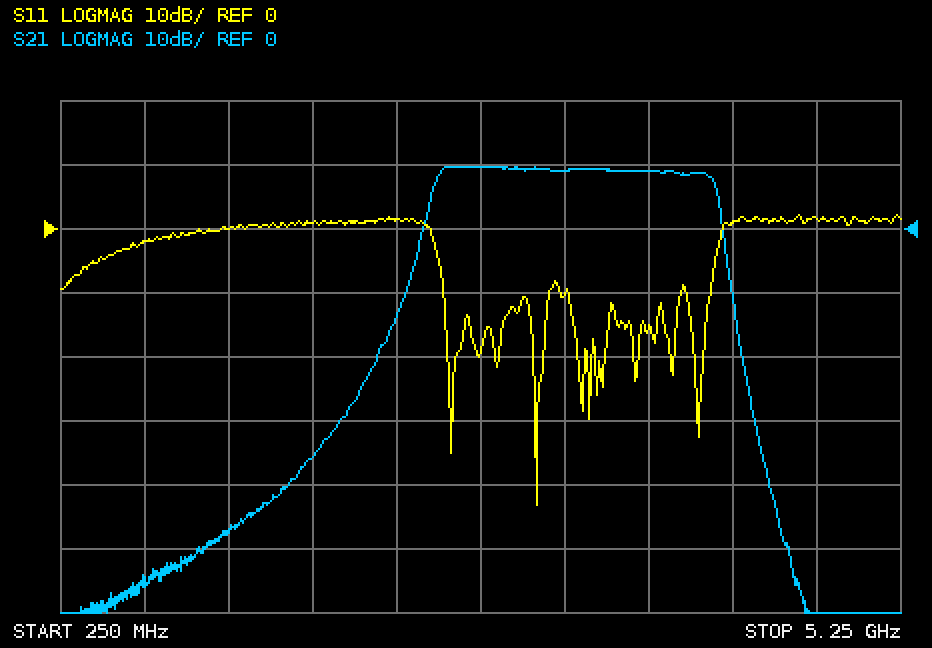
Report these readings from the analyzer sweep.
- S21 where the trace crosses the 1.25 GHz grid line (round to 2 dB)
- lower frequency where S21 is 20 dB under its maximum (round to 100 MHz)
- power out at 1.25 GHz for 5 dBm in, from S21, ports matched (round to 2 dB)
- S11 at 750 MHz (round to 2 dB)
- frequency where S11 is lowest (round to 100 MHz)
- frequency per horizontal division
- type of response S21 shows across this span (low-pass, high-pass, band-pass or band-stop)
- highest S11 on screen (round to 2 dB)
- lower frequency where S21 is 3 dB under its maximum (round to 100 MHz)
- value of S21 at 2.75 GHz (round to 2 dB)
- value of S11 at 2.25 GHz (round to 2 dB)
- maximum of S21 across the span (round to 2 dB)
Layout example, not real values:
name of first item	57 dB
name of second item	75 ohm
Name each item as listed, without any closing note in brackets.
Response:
S21 where the trace crosses the 1.25 GHz grid line	-48 dB
lower frequency where S21 is 20 dB under its maximum	2.3 GHz
power out at 1.25 GHz for 5 dBm in, from S21, ports matched	-42 dBm
S11 at 750 MHz	-2 dB
frequency where S11 is lowest	3.1 GHz
frequency per horizontal division	500 MHz
type of response S21 shows across this span	band-pass
highest S11 on screen	2 dB
lower frequency where S21 is 3 dB under its maximum	2.5 GHz
value of S21 at 2.75 GHz	10 dB
value of S11 at 2.25 GHz	2 dB
maximum of S21 across the span	10 dB
